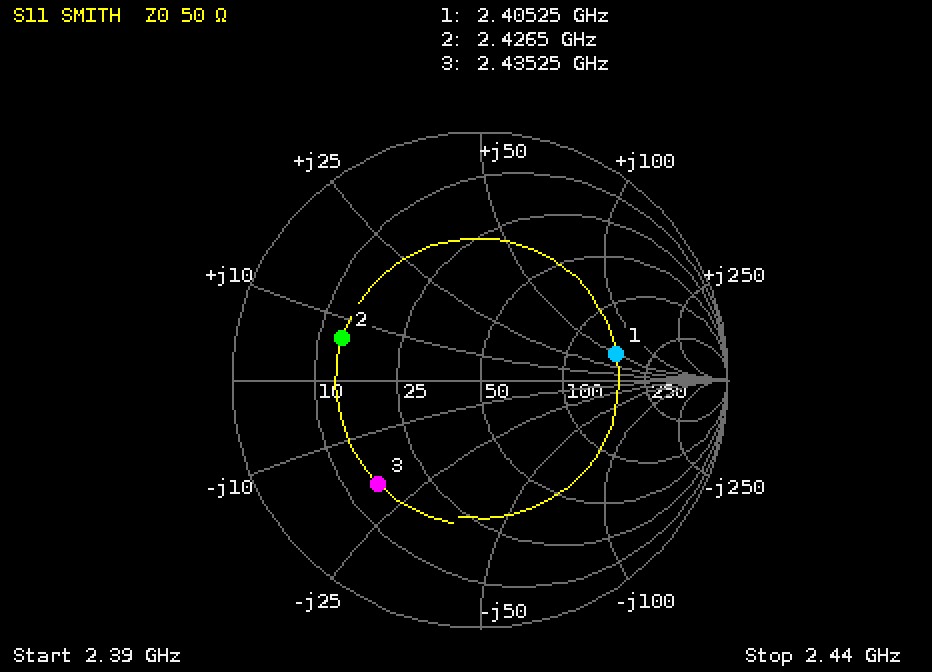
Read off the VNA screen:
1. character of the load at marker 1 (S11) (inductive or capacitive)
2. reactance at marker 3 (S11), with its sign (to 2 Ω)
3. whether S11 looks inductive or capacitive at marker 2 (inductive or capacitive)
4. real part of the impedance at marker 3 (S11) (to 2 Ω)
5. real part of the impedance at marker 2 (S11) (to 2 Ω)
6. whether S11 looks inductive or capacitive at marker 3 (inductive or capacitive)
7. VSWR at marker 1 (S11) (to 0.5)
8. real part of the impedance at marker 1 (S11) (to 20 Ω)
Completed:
inductive
-20 Ω
inductive
16 Ω
14 Ω
capacitive
3.5
160 Ω
